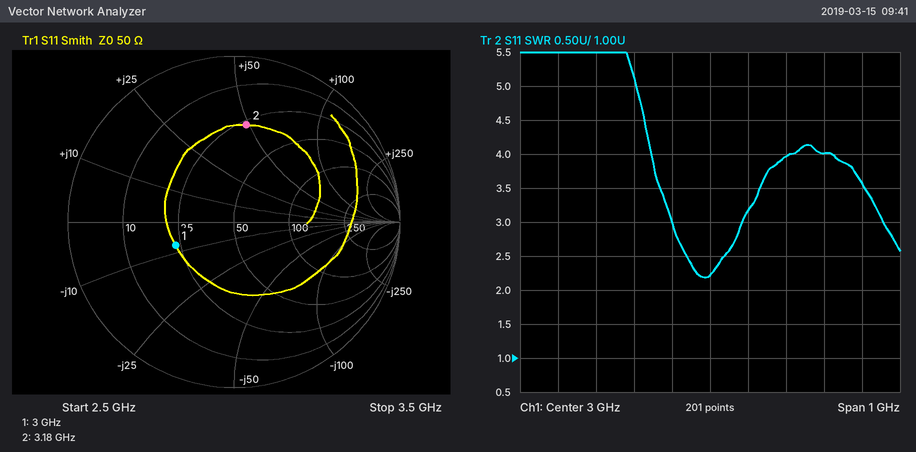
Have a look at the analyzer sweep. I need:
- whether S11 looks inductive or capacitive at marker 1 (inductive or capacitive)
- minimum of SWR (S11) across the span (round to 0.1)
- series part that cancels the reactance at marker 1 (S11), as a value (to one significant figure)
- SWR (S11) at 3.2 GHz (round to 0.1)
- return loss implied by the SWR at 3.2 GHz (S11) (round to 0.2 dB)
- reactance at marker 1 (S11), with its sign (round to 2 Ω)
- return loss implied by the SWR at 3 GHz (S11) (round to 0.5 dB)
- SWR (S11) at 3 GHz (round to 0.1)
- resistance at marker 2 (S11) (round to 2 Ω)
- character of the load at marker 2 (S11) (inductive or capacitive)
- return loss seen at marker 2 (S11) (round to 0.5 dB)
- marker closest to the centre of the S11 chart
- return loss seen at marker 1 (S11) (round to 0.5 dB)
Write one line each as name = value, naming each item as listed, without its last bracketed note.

whether S11 looks inductive or capacitive at marker 1 = capacitive
minimum of SWR (S11) across the span = 2.2
series part that cancels the reactance at marker 1 (S11), as a value = 400 pH
SWR (S11) at 3.2 GHz = 4.0
return loss implied by the SWR at 3.2 GHz (S11) = 4.4 dB
reactance at marker 1 (S11), with its sign = -8 Ω
return loss implied by the SWR at 3 GHz (S11) = 8.5 dB
SWR (S11) at 3 GHz = 2.2
resistance at marker 2 (S11) = 28 Ω
character of the load at marker 2 (S11) = inductive
return loss seen at marker 2 (S11) = 4.5 dB
marker closest to the centre of the S11 chart = marker 1
return loss seen at marker 1 (S11) = 8.5 dB
